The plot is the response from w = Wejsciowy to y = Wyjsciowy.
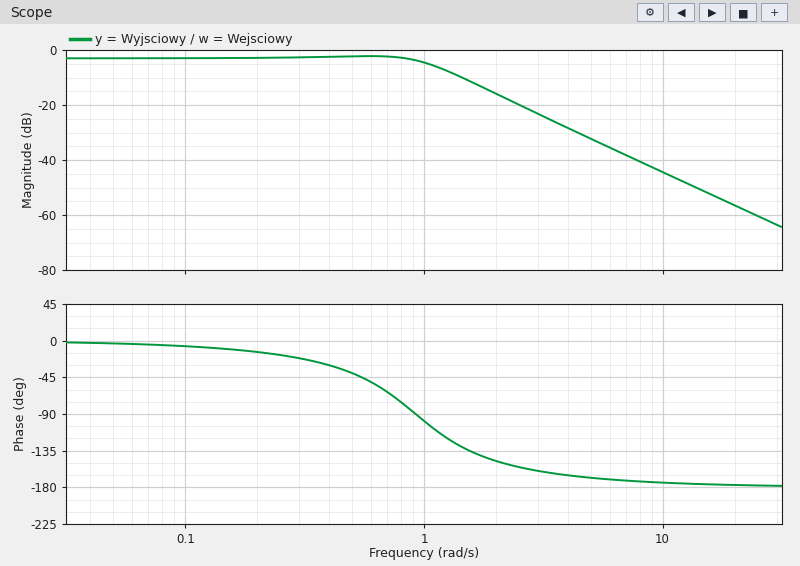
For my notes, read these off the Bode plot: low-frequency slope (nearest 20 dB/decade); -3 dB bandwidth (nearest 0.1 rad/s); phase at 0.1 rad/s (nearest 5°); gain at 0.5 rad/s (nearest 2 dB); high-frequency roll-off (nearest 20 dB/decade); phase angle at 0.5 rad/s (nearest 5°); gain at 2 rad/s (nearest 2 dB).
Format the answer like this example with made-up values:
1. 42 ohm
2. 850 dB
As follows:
1. 0 dB/decade
2. 1.1 rad/s
3. -5°
4. -2 dB
5. -40 dB/decade
6. -40°
7. -16 dB
